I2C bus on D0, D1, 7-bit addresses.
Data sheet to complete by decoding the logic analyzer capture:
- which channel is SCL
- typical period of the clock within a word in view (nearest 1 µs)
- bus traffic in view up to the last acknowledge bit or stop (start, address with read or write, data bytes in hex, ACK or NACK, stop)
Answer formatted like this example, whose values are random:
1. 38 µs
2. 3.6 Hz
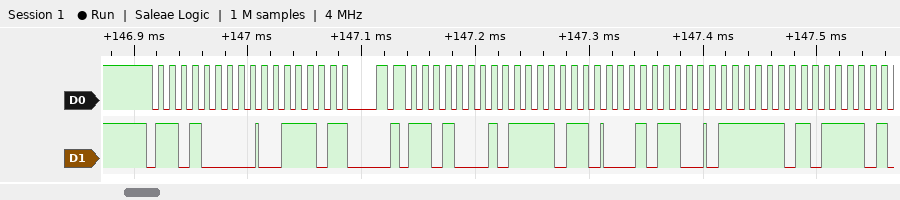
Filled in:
1. D0
2. 10 µs
3. start, address 68 write ACK, 3B ACK, repeated start, address 68 read ACK, F6 ACK, 2C ACK, FD ACK
